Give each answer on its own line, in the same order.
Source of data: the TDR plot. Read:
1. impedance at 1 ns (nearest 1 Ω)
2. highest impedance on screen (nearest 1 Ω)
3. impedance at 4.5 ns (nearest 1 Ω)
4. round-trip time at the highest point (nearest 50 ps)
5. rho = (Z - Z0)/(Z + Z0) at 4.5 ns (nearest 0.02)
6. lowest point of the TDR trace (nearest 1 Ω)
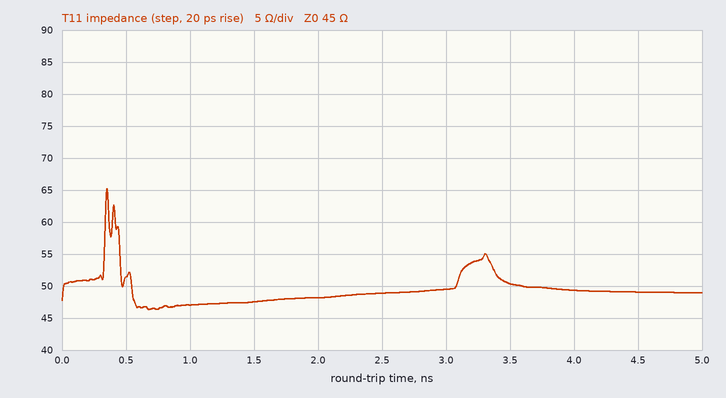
47 Ω
65 Ω
49 Ω
350 ps
+0.04
46 Ω
